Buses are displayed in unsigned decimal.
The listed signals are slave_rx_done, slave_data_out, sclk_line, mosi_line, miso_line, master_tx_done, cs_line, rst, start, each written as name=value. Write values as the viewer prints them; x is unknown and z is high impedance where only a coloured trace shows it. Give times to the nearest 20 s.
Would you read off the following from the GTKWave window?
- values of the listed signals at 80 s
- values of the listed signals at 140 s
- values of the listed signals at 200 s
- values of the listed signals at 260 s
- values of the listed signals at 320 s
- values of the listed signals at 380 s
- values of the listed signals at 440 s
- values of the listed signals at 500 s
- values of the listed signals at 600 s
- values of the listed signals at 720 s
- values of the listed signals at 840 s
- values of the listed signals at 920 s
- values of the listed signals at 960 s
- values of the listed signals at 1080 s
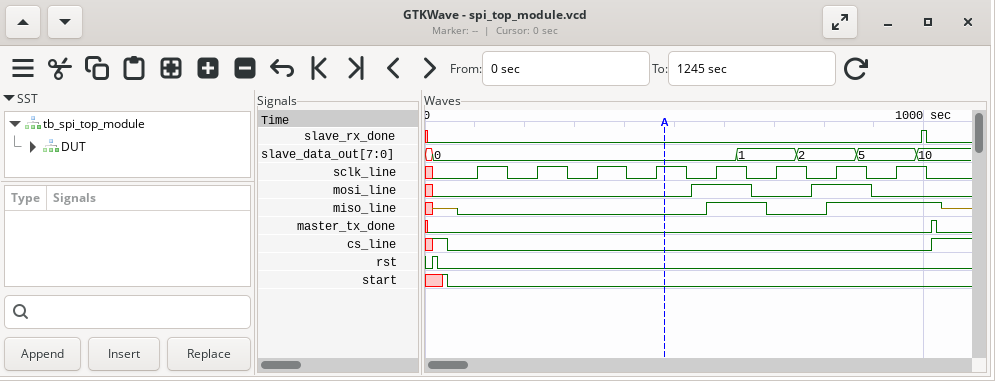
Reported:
slave_rx_done=0, slave_data_out=0, sclk_line=0, mosi_line=0, miso_line=0, master_tx_done=0, cs_line=0, rst=0, start=0
slave_rx_done=0, slave_data_out=0, sclk_line=1, mosi_line=0, miso_line=0, master_tx_done=0, cs_line=0, rst=0, start=0
slave_rx_done=0, slave_data_out=0, sclk_line=0, mosi_line=0, miso_line=0, master_tx_done=0, cs_line=0, rst=0, start=0
slave_rx_done=0, slave_data_out=0, sclk_line=1, mosi_line=0, miso_line=0, master_tx_done=0, cs_line=0, rst=0, start=0
slave_rx_done=0, slave_data_out=0, sclk_line=0, mosi_line=0, miso_line=0, master_tx_done=0, cs_line=0, rst=0, start=0
slave_rx_done=0, slave_data_out=0, sclk_line=1, mosi_line=0, miso_line=0, master_tx_done=0, cs_line=0, rst=0, start=0
slave_rx_done=0, slave_data_out=0, sclk_line=0, mosi_line=0, miso_line=0, master_tx_done=0, cs_line=0, rst=0, start=0
slave_rx_done=0, slave_data_out=0, sclk_line=1, mosi_line=0, miso_line=0, master_tx_done=0, cs_line=0, rst=0, start=0
slave_rx_done=0, slave_data_out=0, sclk_line=1, mosi_line=1, miso_line=1, master_tx_done=0, cs_line=0, rst=0, start=0
slave_rx_done=0, slave_data_out=1, sclk_line=1, mosi_line=0, miso_line=0, master_tx_done=0, cs_line=0, rst=0, start=0
slave_rx_done=0, slave_data_out=2, sclk_line=1, mosi_line=1, miso_line=1, master_tx_done=0, cs_line=0, rst=0, start=0
slave_rx_done=0, slave_data_out=5, sclk_line=0, mosi_line=0, miso_line=1, master_tx_done=0, cs_line=0, rst=0, start=0
slave_rx_done=0, slave_data_out=5, sclk_line=1, mosi_line=0, miso_line=1, master_tx_done=0, cs_line=0, rst=0, start=0
slave_rx_done=0, slave_data_out=10, sclk_line=0, mosi_line=0, miso_line=z, master_tx_done=0, cs_line=1, rst=0, start=0
